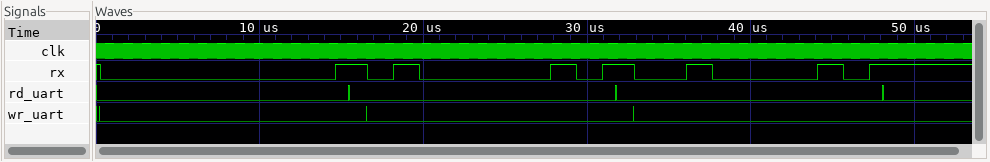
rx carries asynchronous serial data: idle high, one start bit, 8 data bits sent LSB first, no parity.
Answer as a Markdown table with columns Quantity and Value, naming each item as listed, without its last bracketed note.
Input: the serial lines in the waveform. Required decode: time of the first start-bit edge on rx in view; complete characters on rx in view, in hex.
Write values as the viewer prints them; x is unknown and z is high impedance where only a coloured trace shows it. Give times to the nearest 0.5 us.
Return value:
| Quantity | Value |
|---|---|
| time of the first start-bit edge on rx in view | 0 us |
| complete characters on rx in view, in hex | 00, 41, 42 |
